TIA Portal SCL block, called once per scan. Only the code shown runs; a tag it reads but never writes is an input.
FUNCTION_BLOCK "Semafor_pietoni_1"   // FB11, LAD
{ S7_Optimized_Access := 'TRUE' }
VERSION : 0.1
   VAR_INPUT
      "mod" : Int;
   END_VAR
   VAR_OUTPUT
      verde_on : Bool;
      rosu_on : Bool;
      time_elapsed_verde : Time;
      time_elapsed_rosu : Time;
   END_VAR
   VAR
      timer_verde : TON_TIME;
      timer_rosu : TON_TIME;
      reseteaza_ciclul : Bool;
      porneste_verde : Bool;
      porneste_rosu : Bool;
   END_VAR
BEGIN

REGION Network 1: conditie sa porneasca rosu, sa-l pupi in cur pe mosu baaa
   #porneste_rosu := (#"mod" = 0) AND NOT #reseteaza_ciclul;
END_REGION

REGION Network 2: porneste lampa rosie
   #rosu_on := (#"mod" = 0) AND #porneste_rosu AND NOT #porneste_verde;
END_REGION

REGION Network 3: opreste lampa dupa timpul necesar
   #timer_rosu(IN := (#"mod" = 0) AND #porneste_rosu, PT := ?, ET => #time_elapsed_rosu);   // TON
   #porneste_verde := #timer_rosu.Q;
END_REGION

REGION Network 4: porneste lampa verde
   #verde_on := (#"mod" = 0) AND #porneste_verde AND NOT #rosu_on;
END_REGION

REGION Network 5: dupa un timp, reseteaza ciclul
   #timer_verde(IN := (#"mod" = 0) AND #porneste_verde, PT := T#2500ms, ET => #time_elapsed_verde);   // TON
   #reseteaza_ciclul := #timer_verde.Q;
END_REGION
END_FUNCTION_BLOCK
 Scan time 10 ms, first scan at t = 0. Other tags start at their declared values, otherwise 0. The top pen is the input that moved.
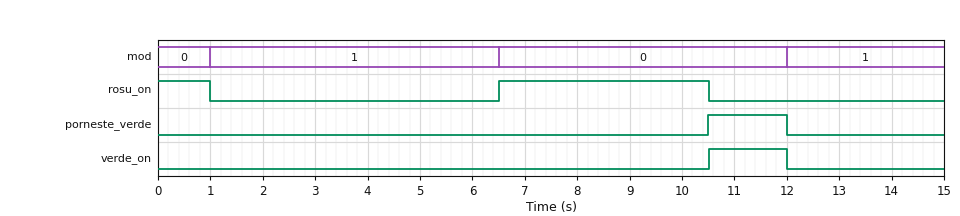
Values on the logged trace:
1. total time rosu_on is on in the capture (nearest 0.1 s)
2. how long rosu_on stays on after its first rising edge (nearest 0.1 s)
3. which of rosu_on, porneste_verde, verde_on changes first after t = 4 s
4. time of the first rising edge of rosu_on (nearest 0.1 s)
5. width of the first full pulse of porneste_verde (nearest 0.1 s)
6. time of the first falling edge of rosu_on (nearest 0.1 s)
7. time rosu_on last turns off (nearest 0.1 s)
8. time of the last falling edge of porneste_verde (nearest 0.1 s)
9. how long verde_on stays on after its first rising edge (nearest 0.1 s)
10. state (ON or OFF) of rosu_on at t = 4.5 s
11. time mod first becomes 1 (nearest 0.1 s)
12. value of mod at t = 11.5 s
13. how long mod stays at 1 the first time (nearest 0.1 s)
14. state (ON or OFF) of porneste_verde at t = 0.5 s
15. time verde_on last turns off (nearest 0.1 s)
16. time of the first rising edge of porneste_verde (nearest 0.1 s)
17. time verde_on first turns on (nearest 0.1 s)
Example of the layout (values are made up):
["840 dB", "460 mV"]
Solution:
["5.0 s", "4.0 s", "rosu_on", "6.5 s", "1.5 s", "1.0 s", "10.5 s", "12.0 s", "1.5 s", "OFF", "1.0 s", "0", "5.5 s", "OFF", "12.0 s", "10.5 s", "10.5 s"]
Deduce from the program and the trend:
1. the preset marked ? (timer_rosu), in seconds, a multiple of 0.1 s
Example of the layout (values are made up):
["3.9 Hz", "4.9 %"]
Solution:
["4.0 s"]
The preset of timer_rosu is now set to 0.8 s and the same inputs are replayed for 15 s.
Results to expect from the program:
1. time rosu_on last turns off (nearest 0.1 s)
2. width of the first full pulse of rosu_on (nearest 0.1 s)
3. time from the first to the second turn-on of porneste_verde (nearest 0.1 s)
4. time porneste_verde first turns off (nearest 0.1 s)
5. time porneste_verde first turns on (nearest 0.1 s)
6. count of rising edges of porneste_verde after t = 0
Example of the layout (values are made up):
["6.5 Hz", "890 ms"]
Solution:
["10.6 s", "0.8 s", "6.5 s", "1.0 s", "0.8 s", "3"]
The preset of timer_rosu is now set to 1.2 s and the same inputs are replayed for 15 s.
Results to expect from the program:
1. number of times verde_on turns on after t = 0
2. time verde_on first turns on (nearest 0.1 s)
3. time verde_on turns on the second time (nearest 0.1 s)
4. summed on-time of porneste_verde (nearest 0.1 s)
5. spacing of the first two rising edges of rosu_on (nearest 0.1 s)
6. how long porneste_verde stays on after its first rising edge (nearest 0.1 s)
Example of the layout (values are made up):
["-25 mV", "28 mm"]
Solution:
["2", "7.7 s", "11.4 s", "3.1 s", "3.7 s", "2.5 s"]
